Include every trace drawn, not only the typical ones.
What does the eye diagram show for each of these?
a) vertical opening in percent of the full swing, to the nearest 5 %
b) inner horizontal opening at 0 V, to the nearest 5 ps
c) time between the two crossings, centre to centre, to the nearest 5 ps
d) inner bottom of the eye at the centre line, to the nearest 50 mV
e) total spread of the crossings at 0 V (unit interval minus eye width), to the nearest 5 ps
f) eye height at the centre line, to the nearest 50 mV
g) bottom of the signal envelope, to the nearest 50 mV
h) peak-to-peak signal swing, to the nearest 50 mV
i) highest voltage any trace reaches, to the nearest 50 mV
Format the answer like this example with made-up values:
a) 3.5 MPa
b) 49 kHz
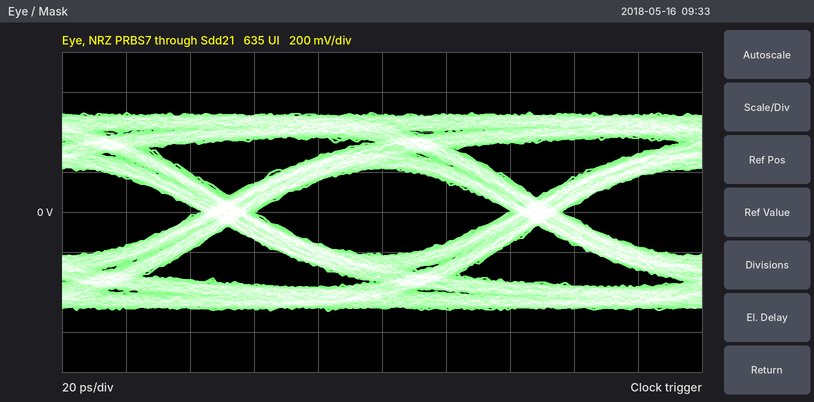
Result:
a) 45 %
b) 80 ps
c) 95 ps
d) -200 mV
e) 15 ps
f) 450 mV
g) -500 mV
h) 1.00 V
i) 500 mV
